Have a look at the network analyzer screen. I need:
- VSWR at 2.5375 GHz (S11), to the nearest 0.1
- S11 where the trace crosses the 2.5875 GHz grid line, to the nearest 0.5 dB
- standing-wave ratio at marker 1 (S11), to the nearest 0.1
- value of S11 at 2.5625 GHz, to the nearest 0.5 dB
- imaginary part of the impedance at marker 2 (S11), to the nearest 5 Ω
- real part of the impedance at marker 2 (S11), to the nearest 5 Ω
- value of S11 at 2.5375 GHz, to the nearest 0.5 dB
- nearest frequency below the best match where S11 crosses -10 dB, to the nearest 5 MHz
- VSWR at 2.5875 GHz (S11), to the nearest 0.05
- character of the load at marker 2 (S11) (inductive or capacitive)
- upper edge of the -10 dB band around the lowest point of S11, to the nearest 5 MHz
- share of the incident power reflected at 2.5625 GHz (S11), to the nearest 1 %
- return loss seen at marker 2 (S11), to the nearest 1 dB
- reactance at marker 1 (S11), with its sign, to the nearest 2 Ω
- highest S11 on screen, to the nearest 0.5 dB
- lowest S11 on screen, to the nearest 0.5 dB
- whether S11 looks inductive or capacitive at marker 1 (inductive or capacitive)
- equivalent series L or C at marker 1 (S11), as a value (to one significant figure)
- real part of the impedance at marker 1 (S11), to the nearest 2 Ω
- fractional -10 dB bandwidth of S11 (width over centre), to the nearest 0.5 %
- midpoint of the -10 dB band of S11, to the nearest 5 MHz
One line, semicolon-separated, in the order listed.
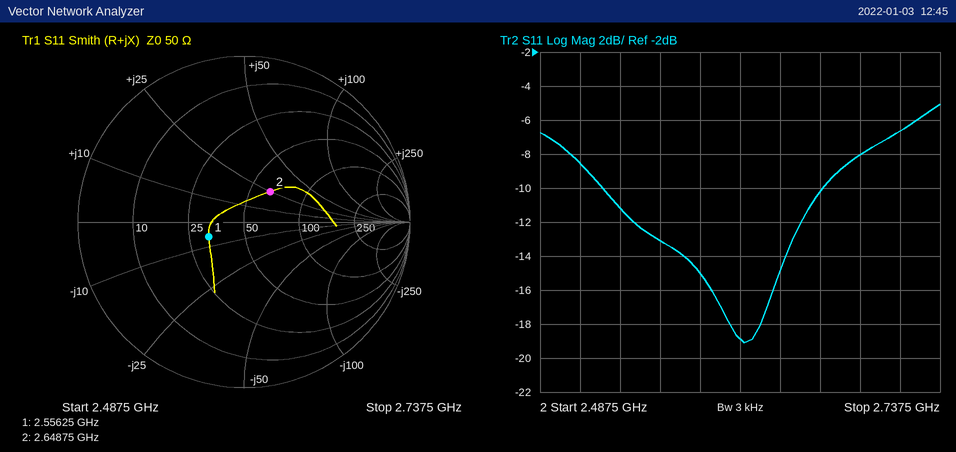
1.8; -15.0 dB; 1.6; -13.0 dB; +25 Ω; 65 Ω; -11.0 dB; 2.525 GHz; 1.45; inductive; 2.665 GHz; 5 %; 12 dB; -6 Ω; -5.0 dB; -19.0 dB; capacitive; 10 pF; 32 Ω; 5.5 %; 2.595 GHz
